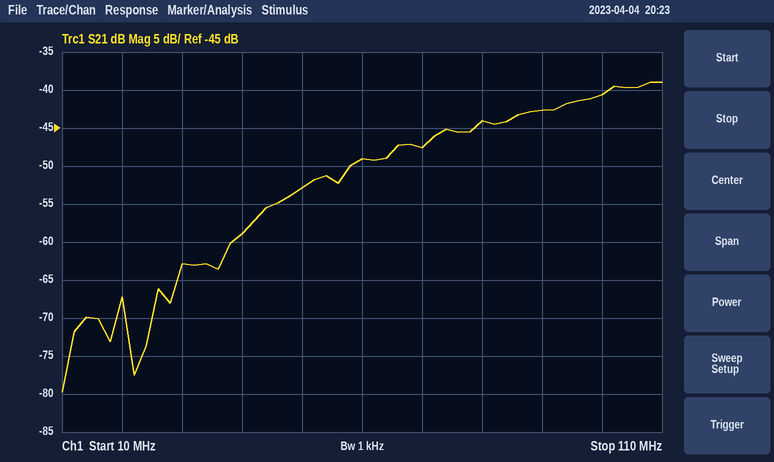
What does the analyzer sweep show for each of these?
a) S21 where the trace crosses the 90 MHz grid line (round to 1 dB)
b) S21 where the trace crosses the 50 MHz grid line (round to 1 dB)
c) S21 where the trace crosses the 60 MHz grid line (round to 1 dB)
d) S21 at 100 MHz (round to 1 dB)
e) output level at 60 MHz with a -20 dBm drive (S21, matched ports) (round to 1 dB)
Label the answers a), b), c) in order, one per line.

a) -43 dB
b) -53 dB
c) -49 dB
d) -41 dB
e) -69 dBm
